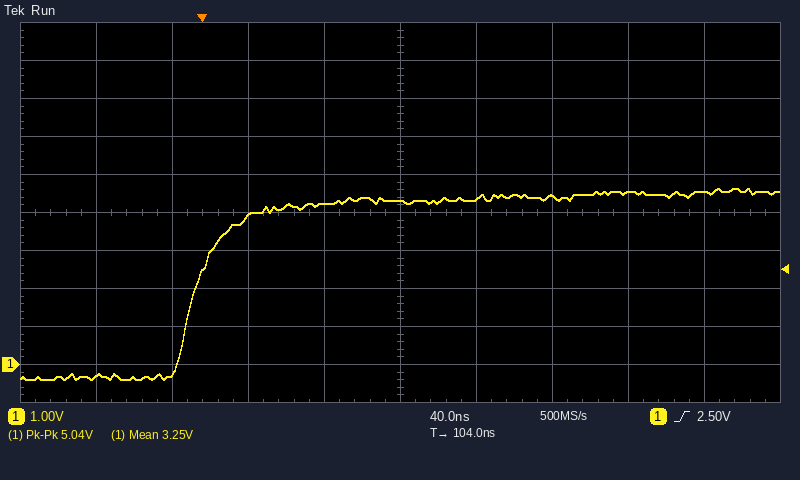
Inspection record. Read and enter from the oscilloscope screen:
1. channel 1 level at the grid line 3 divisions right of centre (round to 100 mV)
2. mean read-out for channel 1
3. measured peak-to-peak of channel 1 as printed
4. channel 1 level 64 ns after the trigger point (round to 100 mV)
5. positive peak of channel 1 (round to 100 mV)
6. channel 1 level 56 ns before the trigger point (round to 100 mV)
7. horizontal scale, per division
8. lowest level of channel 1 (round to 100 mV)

4.5 V
3.25 V
5.04 V
4.2 V
4.6 V
-300 mV
40 ns
-400 mV
